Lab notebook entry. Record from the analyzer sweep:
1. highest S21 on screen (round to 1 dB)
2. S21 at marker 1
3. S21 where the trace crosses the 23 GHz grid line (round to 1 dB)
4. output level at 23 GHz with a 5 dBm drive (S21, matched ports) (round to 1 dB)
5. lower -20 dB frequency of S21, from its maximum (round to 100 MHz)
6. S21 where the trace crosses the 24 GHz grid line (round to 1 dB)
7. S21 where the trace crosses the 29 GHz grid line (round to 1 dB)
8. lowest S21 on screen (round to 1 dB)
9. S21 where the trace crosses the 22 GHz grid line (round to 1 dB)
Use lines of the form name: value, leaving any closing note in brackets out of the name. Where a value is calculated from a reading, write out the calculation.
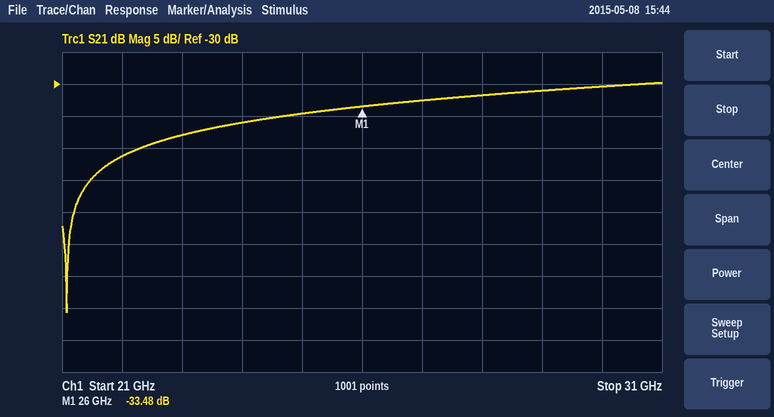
highest S21 on screen: -30 dB
S21 at marker 1: -33.48 dB
S21 where the trace crosses the 23 GHz grid line: -38 dB
output level at 23 GHz with a 5 dBm drive (S21, matched ports): 5 dBm + (-38 dB) = -33 dBm
lower -20 dB frequency of S21, from its maximum: 21.2 GHz
S21 where the trace crosses the 24 GHz grid line: -36 dB
S21 where the trace crosses the 29 GHz grid line: -31 dB
lowest S21 on screen: -66 dB
S21 where the trace crosses the 22 GHz grid line: -41 dB
